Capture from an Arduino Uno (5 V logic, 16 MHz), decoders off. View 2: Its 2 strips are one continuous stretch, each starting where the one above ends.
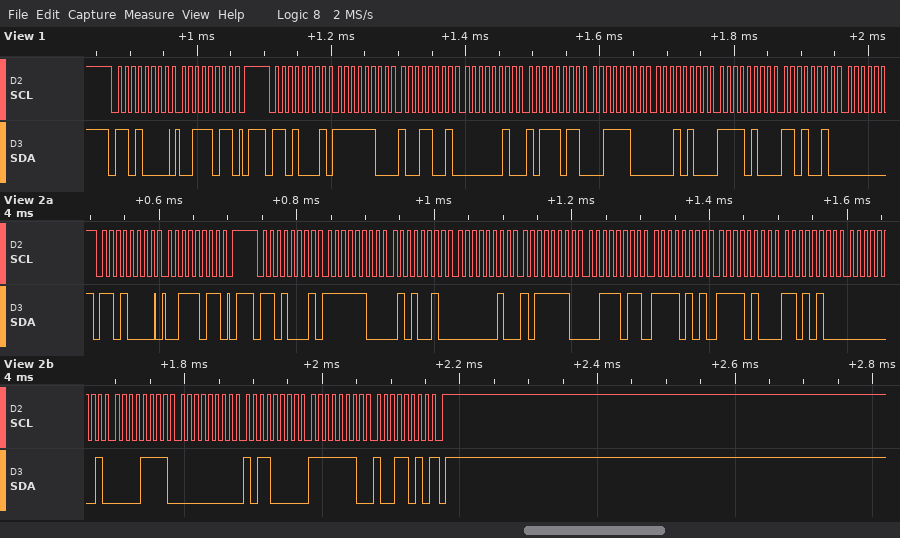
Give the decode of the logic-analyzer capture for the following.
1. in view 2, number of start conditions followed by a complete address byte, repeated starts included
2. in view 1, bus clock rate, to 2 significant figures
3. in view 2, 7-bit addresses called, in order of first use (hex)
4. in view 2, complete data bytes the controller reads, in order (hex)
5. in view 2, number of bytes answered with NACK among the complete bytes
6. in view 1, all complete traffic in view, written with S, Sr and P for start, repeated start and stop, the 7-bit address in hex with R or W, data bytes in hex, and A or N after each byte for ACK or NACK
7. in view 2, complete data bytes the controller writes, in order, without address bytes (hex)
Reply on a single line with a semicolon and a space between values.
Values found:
2; 100 kHz; 0x68; FC 52 02 BE 3B F5 F4 D4 01 0F 00 B0 FE 9A; 1; S 68W A 3B A P S 68R A FC A 99 A 02 A BB A 3C A 14 A F4 A D2 A; 3B
